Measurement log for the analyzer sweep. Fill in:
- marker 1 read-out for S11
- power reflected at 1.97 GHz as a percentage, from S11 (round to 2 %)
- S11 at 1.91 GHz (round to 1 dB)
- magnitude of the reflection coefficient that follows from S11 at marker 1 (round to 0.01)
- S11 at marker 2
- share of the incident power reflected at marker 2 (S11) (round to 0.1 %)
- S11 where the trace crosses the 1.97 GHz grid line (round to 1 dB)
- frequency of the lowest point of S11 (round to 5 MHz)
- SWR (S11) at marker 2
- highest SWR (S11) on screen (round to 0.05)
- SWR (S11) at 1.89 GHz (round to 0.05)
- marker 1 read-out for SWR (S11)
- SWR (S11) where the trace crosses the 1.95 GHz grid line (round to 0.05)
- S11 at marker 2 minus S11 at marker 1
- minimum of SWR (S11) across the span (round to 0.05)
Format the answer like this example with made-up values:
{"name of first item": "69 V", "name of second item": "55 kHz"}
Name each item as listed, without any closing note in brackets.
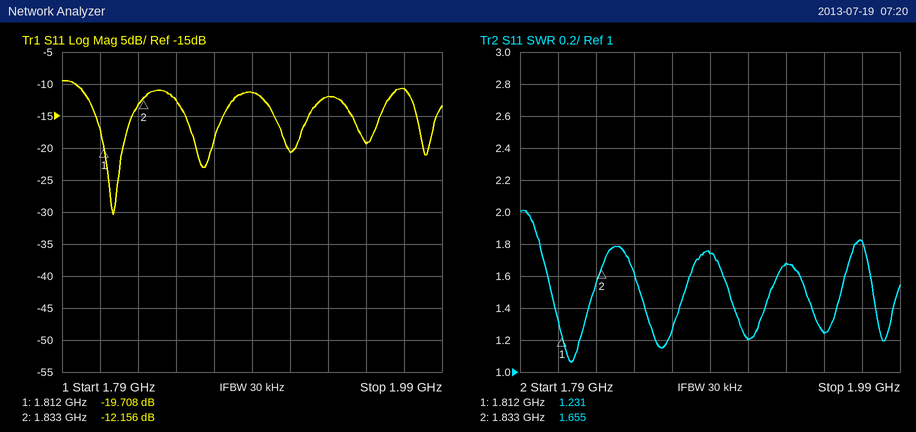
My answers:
{"marker 1 read-out for S11": "-19.708 dB", "power reflected at 1.97 GHz as a percentage, from S11": "8 %", "S11 at 1.91 GHz": "-21 dB", "magnitude of the reflection coefficient that follows from S11 at marker 1": "0.10", "S11 at marker 2": "-12.156 dB", "share of the incident power reflected at marker 2 (S11)": "6.1 %", "S11 where the trace crosses the 1.97 GHz grid line": "-11 dB", "frequency of the lowest point of S11": "1.815 GHz", "SWR (S11) at marker 2": "1.655", "highest SWR (S11) on screen": "2.00", "SWR (S11) at 1.89 GHz": "1.75", "marker 1 read-out for SWR": "1.231", "SWR (S11) where the trace crosses the 1.95 GHz grid line": "1.25", "S11 at marker 2 minus S11 at marker 1": "7.552 dB", "minimum of SWR (S11) across the span": "1.05"}
